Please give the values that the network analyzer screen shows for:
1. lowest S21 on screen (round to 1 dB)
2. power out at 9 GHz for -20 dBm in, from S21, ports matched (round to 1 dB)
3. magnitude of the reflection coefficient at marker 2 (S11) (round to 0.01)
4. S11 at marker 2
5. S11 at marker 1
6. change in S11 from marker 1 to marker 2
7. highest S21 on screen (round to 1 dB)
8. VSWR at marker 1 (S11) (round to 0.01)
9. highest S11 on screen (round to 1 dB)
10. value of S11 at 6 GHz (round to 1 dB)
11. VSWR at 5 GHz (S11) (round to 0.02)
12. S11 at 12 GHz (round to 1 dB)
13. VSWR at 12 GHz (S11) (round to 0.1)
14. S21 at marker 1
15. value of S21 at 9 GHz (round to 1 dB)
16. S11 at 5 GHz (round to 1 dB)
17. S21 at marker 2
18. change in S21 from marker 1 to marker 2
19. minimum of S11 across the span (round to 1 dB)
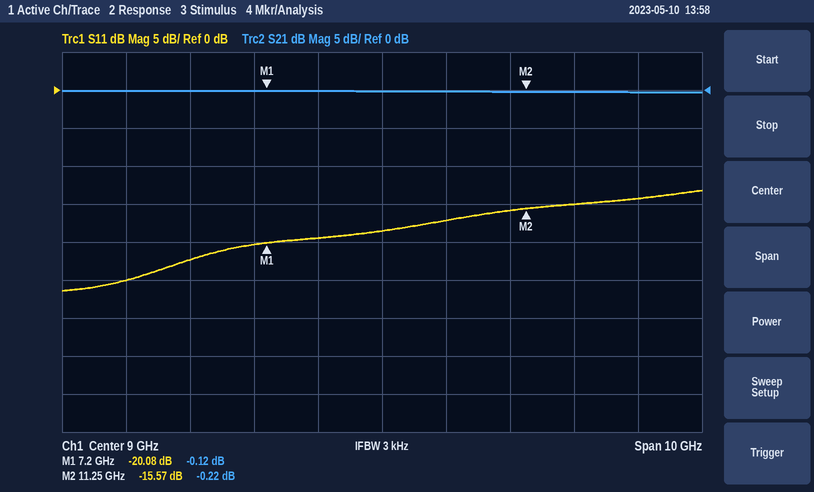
0 dB
-20 dBm
0.17
-15.57 dB
-20.08 dB
4.51 dB
0 dB
1.22
-13 dB
-22 dB
1.12
-15 dB
1.4
-0.12 dB
0 dB
-25 dB
-0.22 dB
-0.10 dB
-26 dB
